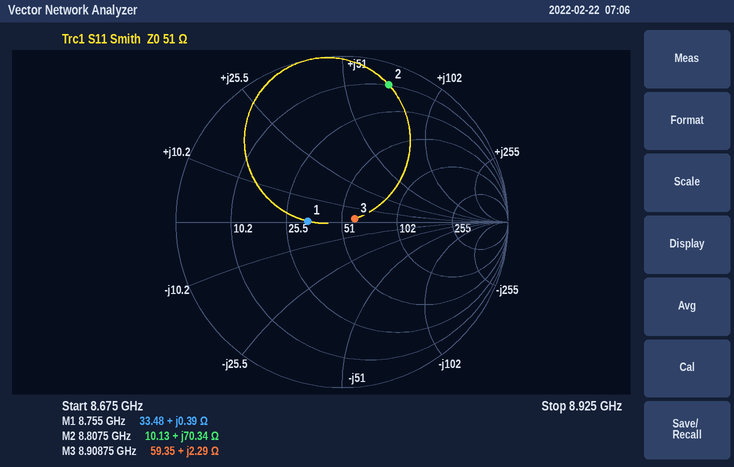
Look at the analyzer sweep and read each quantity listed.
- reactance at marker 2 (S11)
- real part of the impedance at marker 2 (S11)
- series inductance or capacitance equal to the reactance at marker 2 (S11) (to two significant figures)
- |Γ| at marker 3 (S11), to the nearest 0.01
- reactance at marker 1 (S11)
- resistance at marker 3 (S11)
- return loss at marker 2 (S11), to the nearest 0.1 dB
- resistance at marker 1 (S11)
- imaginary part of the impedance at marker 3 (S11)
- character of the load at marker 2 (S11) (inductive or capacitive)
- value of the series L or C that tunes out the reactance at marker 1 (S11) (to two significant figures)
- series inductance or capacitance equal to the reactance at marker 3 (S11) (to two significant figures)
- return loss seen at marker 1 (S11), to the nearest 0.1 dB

+70.34 Ω
10.13 Ω
1.3 nH
0.08
+0.39 Ω
59.35 Ω
1.2 dB
33.48 Ω
+2.29 Ω
inductive
47 pF
41 pH
13.7 dB
